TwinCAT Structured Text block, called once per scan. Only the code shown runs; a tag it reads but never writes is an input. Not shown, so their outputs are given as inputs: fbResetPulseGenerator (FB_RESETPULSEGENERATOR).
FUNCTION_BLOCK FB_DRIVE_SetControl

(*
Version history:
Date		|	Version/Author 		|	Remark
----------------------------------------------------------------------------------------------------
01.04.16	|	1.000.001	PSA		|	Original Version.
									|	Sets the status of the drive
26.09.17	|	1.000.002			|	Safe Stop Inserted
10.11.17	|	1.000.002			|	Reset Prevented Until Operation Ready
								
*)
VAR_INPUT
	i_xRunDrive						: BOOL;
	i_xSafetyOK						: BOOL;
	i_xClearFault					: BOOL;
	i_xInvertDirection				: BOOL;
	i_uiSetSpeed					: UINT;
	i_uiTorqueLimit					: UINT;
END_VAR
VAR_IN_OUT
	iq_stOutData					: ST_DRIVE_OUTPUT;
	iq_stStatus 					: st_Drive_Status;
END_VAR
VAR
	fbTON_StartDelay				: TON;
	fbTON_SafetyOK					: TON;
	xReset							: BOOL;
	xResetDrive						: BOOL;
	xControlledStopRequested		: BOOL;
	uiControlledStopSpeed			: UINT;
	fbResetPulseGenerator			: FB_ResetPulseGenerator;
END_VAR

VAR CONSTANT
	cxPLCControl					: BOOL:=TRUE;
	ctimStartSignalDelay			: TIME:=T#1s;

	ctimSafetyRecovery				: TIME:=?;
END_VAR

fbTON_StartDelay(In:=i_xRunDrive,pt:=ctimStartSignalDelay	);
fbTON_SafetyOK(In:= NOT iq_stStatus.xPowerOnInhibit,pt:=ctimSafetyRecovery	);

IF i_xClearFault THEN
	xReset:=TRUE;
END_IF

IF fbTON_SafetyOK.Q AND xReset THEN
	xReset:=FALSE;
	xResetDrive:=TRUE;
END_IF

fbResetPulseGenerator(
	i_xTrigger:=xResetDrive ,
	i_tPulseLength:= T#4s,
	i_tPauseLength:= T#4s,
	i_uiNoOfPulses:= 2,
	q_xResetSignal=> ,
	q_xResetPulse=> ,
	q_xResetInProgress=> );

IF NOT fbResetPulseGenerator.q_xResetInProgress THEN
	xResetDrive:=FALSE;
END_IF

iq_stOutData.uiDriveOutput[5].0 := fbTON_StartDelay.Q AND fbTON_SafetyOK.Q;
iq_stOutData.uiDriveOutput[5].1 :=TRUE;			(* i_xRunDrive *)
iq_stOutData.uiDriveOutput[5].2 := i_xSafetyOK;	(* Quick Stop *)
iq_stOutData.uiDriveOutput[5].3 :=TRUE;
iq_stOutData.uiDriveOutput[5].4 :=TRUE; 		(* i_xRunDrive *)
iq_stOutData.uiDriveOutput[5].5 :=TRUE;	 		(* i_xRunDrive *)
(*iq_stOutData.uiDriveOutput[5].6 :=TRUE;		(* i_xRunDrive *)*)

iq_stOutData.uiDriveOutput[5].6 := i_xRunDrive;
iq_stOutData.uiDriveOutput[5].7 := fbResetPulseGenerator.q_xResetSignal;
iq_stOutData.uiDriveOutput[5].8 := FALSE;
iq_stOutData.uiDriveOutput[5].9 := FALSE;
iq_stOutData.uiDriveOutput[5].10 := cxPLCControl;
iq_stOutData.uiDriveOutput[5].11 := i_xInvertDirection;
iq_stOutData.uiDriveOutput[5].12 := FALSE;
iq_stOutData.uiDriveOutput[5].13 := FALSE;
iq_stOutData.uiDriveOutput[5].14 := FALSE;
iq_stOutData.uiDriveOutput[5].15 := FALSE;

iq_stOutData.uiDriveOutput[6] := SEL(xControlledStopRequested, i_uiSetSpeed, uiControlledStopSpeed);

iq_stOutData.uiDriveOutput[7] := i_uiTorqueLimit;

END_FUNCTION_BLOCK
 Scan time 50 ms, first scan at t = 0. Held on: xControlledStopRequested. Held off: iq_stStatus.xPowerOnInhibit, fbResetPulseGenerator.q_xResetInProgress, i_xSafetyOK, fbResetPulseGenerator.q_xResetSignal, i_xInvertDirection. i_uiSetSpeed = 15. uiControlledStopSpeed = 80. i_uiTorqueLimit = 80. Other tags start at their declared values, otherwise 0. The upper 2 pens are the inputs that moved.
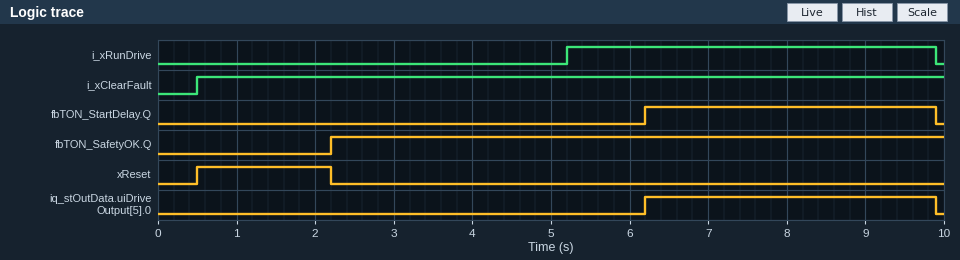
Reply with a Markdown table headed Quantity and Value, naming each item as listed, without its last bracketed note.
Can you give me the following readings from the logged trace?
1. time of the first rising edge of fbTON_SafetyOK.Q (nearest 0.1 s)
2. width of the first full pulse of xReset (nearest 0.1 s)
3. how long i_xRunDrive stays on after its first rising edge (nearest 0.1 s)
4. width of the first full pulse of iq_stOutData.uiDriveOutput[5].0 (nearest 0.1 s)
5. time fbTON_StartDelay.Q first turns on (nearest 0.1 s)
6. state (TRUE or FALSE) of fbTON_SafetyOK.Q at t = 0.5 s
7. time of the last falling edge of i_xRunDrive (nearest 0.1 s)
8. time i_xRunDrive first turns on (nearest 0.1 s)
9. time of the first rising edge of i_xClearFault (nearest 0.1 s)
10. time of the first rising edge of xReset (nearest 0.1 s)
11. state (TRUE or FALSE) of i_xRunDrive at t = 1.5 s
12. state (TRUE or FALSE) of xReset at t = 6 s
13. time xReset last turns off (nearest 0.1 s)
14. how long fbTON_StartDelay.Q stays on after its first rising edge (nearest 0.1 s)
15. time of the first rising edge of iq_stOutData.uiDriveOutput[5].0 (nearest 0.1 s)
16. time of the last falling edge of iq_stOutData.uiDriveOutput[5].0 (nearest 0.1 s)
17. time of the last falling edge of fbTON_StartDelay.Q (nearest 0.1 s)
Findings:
| Quantity | Value |
|---|---|
| time of the first rising edge of fbTON_SafetyOK.Q | 2.2 s |
| width of the first full pulse of xReset | 1.7 s |
| how long i_xRunDrive stays on after its first rising edge | 4.7 s |
| width of the first full pulse of iq_stOutData.uiDriveOutput[5].0 | 3.7 s |
| time fbTON_StartDelay.Q first turns on | 6.2 s |
| state (TRUE or FALSE) of fbTON_SafetyOK.Q at t = 0.5 s | FALSE |
| time of the last falling edge of i_xRunDrive | 9.9 s |
| time i_xRunDrive first turns on | 5.2 s |
| time of the first rising edge of i_xClearFault | 0.5 s |
| time of the first rising edge of xReset | 0.5 s |
| state (TRUE or FALSE) of i_xRunDrive at t = 1.5 s | FALSE |
| state (TRUE or FALSE) of xReset at t = 6 s | FALSE |
| time xReset last turns off | 2.2 s |
| how long fbTON_StartDelay.Q stays on after its first rising edge | 3.7 s |
| time of the first rising edge of iq_stOutData.uiDriveOutput[5].0 | 6.2 s |
| time of the last falling edge of iq_stOutData.uiDriveOutput[5].0 | 9.9 s |
| time of the last falling edge of fbTON_StartDelay.Q | 9.9 s |
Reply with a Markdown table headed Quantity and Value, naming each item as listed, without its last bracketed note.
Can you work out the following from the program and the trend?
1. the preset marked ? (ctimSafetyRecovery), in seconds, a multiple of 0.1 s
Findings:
| Quantity | Value |
|---|---|
| the preset marked ? (ctimSafetyRecovery), in seconds, a multiple of 0.1 s | 2.2 s |
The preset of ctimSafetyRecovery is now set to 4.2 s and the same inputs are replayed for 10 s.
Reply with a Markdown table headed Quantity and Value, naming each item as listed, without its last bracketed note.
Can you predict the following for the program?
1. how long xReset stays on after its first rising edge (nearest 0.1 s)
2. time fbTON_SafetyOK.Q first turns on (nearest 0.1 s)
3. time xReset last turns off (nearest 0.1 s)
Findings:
| Quantity | Value |
|---|---|
| how long xReset stays on after its first rising edge | 3.7 s |
| time fbTON_SafetyOK.Q first turns on | 4.2 s |
| time xReset last turns off | 4.2 s |
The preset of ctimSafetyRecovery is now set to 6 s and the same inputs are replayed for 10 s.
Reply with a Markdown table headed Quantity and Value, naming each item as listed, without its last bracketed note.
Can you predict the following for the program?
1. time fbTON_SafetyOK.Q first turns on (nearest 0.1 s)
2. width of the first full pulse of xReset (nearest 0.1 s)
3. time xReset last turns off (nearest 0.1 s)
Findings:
| Quantity | Value |
|---|---|
| time fbTON_SafetyOK.Q first turns on | 6.0 s |
| width of the first full pulse of xReset | 5.5 s |
| time xReset last turns off | 6.0 s |
